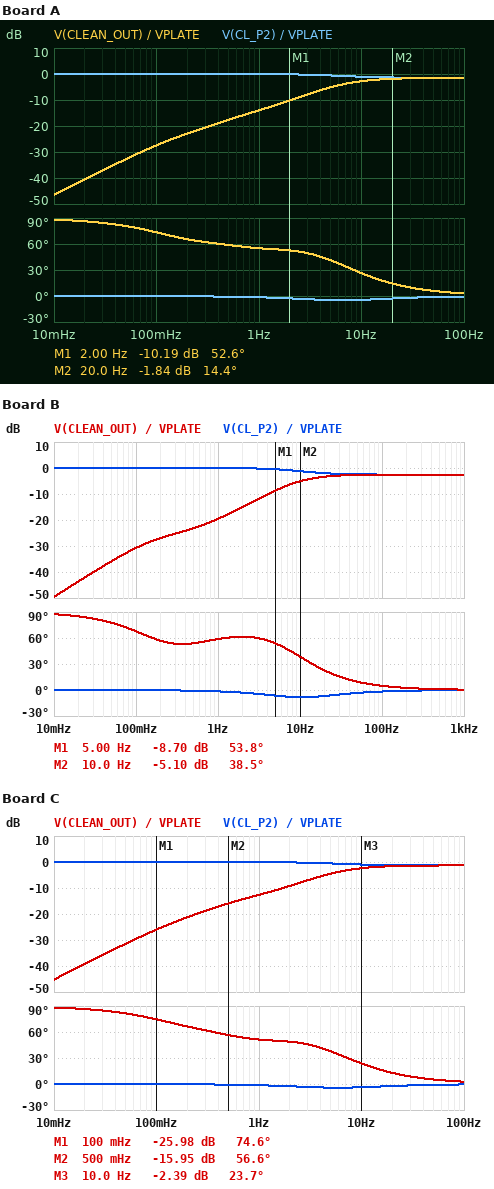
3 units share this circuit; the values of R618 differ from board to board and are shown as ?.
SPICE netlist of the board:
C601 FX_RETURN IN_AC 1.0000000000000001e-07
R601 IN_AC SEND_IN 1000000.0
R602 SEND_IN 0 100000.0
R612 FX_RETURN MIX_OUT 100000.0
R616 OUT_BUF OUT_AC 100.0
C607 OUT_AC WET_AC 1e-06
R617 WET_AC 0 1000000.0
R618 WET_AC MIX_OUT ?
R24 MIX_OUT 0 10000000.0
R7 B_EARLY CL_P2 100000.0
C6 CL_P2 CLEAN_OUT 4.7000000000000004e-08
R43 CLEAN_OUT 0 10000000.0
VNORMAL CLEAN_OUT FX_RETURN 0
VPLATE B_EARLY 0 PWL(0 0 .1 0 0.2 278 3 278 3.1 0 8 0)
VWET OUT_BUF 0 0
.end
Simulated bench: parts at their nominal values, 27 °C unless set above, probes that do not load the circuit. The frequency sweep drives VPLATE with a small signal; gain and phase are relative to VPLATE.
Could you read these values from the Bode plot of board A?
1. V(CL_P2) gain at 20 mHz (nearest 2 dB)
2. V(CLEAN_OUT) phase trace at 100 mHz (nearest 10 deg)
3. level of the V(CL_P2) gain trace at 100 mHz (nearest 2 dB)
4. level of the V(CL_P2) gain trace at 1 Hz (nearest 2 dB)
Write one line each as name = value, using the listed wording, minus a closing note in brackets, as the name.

V(CL_P2) gain at 20 mHz = 0 dB
V(CLEAN_OUT) phase trace at 100 mHz = 70 deg
level of the V(CL_P2) gain trace at 100 mHz = 0 dB
level of the V(CL_P2) gain trace at 1 Hz = 0 dB
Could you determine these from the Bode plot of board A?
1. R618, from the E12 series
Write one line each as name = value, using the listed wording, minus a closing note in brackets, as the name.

R618, from the E12 series = 1.2 MΩ
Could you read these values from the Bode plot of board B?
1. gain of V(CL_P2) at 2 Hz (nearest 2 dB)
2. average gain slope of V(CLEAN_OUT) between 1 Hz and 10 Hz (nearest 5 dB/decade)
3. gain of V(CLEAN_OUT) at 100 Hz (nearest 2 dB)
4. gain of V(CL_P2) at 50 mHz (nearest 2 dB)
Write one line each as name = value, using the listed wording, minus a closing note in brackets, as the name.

gain of V(CL_P2) at 2 Hz = 0 dB
average gain slope of V(CLEAN_OUT) between 1 Hz and 10 Hz = 15 dB/decade
gain of V(CLEAN_OUT) at 100 Hz = -2 dB
gain of V(CL_P2) at 50 mHz = 0 dB
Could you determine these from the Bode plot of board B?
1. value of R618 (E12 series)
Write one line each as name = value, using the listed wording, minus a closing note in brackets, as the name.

value of R618 = 330 kΩ
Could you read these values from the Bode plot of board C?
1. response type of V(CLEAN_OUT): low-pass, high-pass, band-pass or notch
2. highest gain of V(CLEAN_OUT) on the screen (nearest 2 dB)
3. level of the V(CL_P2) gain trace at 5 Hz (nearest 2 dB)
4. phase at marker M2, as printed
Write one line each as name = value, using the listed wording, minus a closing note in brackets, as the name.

response type of V(CLEAN_OUT): low-pass, high-pass, band-pass or notch = high-pass
highest gain of V(CLEAN_OUT) on the screen = -2 dB
level of the V(CL_P2) gain trace at 5 Hz = 0 dB
phase at marker M2, as printed = 56.6 deg
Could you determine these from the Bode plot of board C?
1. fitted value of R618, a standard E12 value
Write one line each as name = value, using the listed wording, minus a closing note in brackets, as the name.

fitted value of R618, a standard E12 value = 1.8 MΩ
